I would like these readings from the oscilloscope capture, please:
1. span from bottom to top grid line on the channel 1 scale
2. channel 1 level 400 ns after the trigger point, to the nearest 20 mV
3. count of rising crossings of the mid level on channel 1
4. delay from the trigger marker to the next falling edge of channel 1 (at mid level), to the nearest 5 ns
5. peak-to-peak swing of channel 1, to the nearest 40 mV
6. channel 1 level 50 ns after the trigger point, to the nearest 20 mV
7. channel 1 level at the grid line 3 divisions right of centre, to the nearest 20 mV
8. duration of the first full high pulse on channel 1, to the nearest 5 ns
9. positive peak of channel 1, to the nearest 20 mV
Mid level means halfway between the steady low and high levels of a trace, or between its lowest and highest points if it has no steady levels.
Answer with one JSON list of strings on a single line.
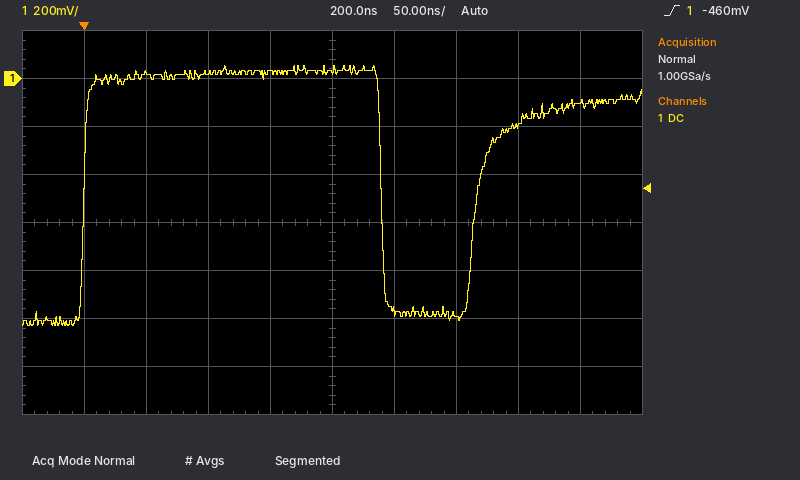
["1.6 V", "-100 mV", "2", "240 ns", "1.08 V", "20 mV", "-200 mV", "240 ns", "60 mV"]
